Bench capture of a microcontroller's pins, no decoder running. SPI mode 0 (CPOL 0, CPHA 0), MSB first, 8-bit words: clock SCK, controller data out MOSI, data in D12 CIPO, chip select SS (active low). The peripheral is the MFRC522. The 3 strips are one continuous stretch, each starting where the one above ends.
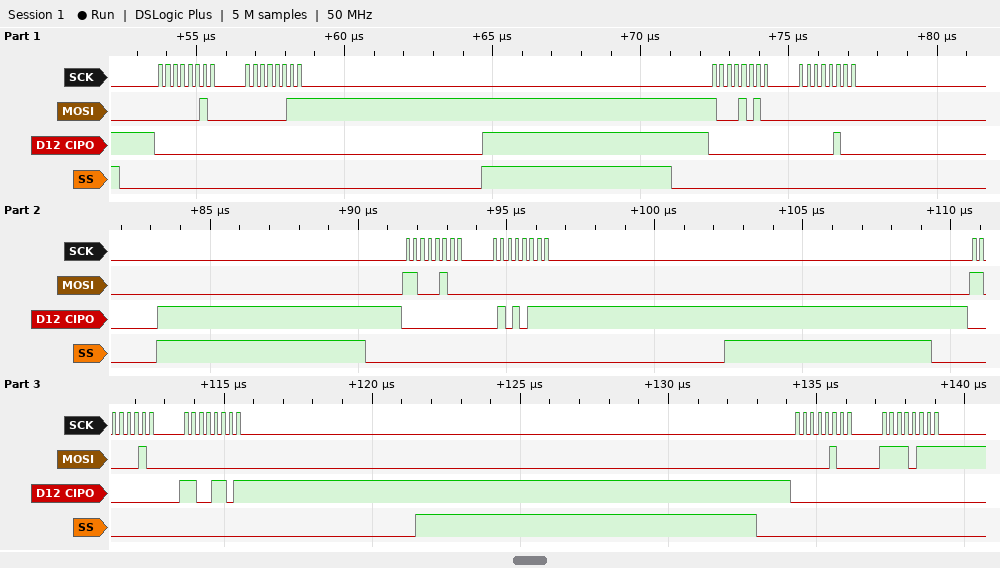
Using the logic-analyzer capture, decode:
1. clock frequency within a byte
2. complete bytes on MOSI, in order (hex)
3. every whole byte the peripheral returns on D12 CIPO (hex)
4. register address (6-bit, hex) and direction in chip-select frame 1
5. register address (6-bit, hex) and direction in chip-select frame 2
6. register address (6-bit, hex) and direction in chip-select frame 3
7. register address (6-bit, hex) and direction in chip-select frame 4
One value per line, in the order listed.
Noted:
4 MHz
02 03 8A 00 C4 00 C2 00 04 F7
00 00 00 04 00 57 00 CD 00 00
0x01 write
0x05 read
0x22 read
0x21 read
